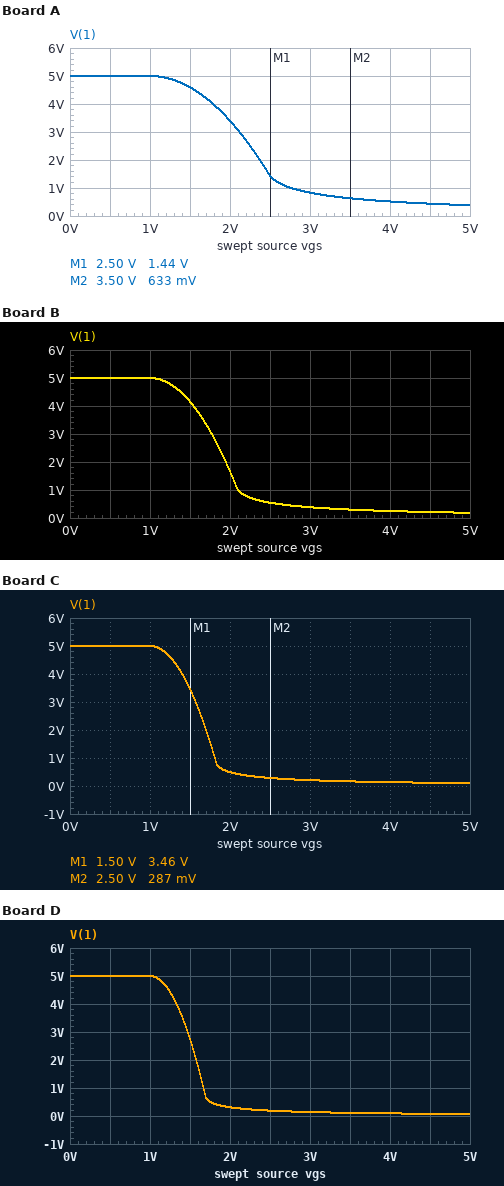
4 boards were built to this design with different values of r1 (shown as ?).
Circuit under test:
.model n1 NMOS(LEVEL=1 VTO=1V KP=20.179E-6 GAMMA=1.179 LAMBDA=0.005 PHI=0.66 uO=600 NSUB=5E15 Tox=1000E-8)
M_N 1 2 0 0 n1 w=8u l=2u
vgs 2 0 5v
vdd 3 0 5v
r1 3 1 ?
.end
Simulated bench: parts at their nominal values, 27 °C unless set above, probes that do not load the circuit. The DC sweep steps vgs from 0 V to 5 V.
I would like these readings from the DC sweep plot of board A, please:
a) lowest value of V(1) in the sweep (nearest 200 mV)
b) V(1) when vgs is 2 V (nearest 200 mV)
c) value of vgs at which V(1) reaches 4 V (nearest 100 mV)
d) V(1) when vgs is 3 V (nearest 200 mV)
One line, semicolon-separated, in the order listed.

400 mV; 3.4 V; 1.8 V; 800 mV
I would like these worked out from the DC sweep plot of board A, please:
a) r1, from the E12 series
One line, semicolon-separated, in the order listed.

39 kΩ
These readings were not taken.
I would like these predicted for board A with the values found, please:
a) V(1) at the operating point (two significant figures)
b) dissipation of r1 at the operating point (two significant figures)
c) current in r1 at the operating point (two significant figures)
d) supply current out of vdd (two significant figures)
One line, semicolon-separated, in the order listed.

380 mV; 550 µW; 120 µA; 120 µA
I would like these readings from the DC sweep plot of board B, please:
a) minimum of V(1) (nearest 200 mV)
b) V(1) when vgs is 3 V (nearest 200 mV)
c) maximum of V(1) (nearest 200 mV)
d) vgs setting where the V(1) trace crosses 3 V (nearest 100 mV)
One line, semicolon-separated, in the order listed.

200 mV; 400 mV; 5.0 V; 1.8 V
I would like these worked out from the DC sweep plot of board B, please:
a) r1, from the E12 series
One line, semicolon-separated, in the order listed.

82 kΩ
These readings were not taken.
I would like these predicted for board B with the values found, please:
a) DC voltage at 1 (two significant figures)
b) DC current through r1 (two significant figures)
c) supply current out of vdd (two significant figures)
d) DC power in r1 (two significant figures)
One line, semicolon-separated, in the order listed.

190 mV; 59 µA; 59 µA; 280 µW
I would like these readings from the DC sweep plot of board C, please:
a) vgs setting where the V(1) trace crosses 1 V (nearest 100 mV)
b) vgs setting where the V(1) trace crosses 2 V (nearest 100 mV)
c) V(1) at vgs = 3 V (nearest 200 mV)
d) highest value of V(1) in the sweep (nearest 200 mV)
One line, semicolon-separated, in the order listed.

1.8 V; 1.7 V; 200 mV; 5.0 V
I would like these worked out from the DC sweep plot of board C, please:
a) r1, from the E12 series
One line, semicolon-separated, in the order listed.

150 kΩ
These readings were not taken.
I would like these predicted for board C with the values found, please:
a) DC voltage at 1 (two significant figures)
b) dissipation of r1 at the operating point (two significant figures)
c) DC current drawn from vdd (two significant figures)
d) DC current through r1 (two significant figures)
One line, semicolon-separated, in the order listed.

100 mV; 160 µW; 33 µA; 33 µA
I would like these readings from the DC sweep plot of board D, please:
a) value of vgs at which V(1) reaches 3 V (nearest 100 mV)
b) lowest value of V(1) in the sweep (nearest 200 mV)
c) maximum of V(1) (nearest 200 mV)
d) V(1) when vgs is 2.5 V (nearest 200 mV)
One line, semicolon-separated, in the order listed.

1.5 V; 0 V; 5.0 V; 200 mV
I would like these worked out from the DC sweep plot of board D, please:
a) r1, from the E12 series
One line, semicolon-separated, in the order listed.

220 kΩ
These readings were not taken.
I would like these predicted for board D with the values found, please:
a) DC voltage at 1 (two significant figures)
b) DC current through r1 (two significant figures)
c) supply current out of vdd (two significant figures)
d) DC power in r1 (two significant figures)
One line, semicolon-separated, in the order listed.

70 mV; 22 µA; 22 µA; 110 µW
